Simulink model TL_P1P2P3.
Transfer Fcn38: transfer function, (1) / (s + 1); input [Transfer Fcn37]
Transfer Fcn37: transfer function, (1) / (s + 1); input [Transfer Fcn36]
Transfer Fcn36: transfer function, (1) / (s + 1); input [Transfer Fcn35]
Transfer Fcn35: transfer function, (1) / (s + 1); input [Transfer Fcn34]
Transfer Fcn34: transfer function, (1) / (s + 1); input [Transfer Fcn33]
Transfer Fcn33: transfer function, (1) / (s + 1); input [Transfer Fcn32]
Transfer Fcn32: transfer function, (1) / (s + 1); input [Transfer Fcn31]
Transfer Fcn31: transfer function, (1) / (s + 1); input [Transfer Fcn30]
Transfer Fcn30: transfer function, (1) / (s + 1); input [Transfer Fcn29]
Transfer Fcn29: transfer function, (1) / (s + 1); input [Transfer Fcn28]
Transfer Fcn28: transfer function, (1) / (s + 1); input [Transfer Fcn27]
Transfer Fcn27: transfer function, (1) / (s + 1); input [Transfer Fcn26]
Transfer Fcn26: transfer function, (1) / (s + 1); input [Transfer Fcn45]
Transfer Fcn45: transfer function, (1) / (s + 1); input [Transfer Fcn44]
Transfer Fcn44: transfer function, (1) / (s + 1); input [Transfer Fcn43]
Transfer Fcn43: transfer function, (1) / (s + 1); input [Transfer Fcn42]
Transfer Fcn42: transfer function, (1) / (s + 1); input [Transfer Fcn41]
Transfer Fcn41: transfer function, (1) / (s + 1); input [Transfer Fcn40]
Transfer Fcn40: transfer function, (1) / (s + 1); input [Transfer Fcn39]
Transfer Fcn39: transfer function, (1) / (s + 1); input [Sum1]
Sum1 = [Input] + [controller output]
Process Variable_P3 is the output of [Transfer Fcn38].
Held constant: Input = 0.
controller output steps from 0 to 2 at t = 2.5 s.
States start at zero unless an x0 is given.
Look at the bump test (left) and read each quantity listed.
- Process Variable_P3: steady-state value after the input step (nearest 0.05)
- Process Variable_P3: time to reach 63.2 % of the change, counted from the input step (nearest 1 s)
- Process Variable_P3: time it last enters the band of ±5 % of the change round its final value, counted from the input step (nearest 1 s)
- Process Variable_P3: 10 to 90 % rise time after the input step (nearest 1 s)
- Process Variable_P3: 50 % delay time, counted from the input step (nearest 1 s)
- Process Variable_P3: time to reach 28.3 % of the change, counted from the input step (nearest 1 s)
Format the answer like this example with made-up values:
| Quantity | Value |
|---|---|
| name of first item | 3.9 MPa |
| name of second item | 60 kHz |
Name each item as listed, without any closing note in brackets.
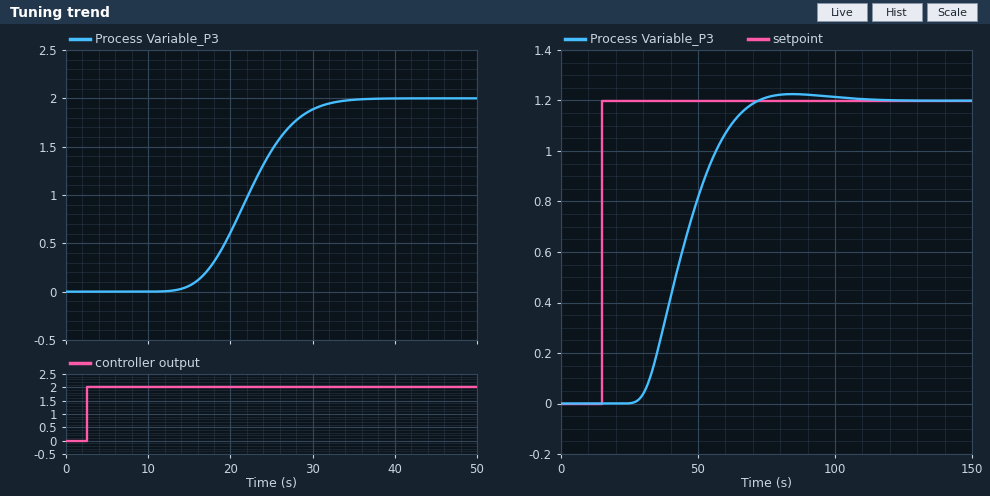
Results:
| Quantity | Value |
|---|---|
| Process Variable_P3: steady-state value after the input step | 2.00 |
| Process Variable_P3: time to reach 63.2 % of the change, counted from the input step | 21 s |
| Process Variable_P3: time it last enters the band of ±5 % of the change round its final value, counted from the input step | 28 s |
| Process Variable_P3: 10 to 90 % rise time after the input step | 11 s |
| Process Variable_P3: 50 % delay time, counted from the input step | 20 s |
| Process Variable_P3: time to reach 28.3 % of the change, counted from the input step | 17 s |
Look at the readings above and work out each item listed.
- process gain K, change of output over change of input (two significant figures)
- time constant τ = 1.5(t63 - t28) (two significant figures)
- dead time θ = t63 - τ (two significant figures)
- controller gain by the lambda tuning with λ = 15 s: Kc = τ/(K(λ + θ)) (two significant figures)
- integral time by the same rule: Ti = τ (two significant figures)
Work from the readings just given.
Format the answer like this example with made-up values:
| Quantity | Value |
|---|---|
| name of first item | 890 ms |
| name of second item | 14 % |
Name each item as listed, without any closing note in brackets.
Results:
| Quantity | Value |
|---|---|
| process gain K, change of output over change of input | 1.0 |
| time constant τ = 1.5(t63 - t28) | 6.0 s |
| dead time θ = t63 - τ | 15 s |
| controller gain by the lambda tuning with λ = 15 s: Kc = τ/(K(λ + θ)) | 0.20 |
| integral time by the same rule: Ti = τ | 6.0 s |
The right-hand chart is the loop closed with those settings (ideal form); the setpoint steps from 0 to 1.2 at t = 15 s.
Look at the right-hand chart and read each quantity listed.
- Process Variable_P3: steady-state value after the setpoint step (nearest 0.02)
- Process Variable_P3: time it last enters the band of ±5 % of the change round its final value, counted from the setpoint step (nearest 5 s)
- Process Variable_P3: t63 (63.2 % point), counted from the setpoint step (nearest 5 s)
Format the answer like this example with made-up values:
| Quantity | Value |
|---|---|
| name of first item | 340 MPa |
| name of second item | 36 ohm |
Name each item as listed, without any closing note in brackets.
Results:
| Quantity | Value |
|---|---|
| Process Variable_P3: steady-state value after the setpoint step | 1.20 |
| Process Variable_P3: time it last enters the band of ±5 % of the change round its final value, counted from the setpoint step | 50 s |
| Process Variable_P3: t63 (63.2 % point), counted from the setpoint step | 35 s |
